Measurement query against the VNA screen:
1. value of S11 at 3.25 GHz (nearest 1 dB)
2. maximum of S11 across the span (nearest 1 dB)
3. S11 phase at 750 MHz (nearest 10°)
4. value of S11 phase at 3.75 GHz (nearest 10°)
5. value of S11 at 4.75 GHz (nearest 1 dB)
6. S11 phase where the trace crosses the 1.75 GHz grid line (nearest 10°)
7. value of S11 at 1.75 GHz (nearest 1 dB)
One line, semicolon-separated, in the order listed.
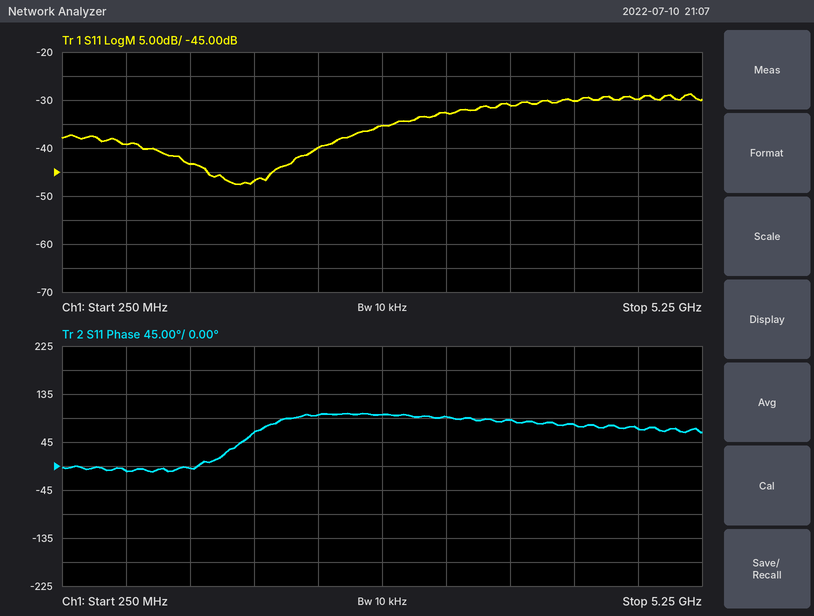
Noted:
-33 dB; -29 dB; -10°; 90°; -30 dB; 60°; -47 dB
